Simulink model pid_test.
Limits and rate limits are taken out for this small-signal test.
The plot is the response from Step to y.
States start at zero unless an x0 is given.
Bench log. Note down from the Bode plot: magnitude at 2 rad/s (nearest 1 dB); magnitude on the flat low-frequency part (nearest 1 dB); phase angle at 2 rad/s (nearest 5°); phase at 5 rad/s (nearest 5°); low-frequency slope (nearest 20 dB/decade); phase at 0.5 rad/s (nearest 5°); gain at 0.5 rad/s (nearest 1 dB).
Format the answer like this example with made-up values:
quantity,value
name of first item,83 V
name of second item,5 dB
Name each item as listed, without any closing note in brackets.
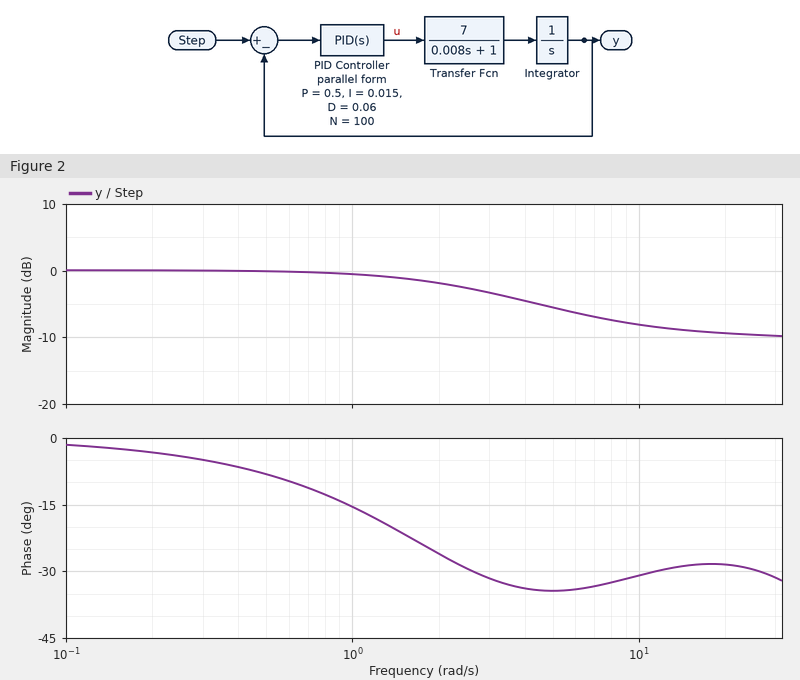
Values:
quantity,value
magnitude at 2 rad/s,-2 dB
magnitude on the flat low-frequency part,0 dB
phase angle at 2 rad/s,-25°
phase at 5 rad/s,-35°
low-frequency slope,0 dB/decade
phase at 0.5 rad/s,-10°
gain at 0.5 rad/s,0 dB
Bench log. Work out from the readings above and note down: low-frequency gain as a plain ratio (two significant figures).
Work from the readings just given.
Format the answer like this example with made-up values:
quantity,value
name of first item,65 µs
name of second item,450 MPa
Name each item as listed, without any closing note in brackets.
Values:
quantity,value
low-frequency gain as a plain ratio,1.0
